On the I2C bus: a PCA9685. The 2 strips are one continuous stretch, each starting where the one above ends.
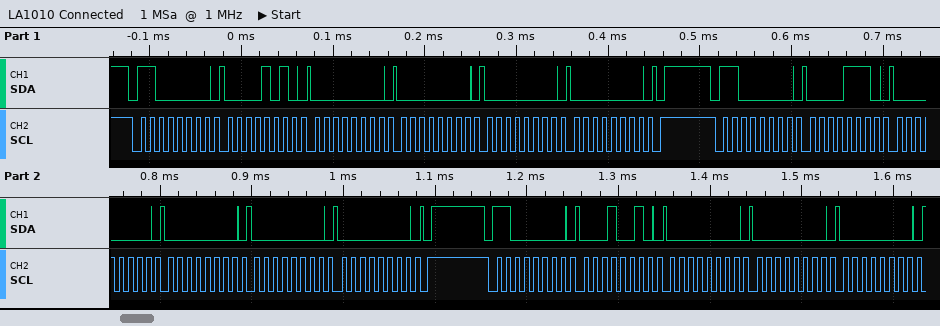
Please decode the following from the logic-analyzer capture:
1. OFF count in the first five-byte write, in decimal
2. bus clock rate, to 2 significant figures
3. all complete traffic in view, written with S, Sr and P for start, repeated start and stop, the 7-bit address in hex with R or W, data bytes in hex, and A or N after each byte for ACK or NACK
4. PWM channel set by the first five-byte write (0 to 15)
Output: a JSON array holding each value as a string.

["0", "100 kHz", "S 60W A 0A A 00 A 00 A 00 A 00 A P S 60W A 0E A 00 A 00 A 00 A 00 A P S 60W A 12 A 00 A 00 A 00 A", "1"]
